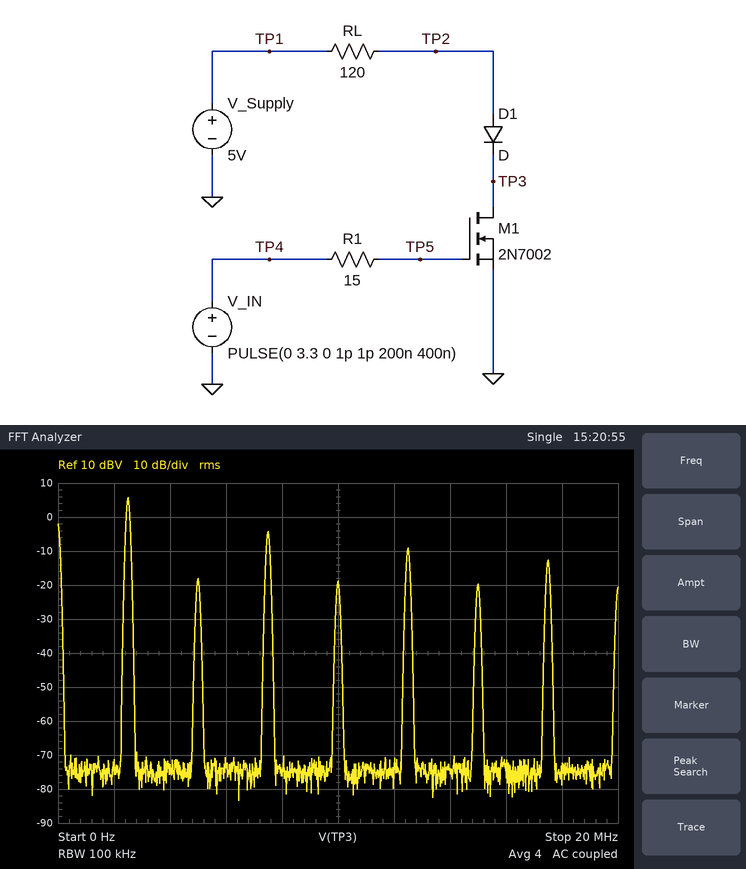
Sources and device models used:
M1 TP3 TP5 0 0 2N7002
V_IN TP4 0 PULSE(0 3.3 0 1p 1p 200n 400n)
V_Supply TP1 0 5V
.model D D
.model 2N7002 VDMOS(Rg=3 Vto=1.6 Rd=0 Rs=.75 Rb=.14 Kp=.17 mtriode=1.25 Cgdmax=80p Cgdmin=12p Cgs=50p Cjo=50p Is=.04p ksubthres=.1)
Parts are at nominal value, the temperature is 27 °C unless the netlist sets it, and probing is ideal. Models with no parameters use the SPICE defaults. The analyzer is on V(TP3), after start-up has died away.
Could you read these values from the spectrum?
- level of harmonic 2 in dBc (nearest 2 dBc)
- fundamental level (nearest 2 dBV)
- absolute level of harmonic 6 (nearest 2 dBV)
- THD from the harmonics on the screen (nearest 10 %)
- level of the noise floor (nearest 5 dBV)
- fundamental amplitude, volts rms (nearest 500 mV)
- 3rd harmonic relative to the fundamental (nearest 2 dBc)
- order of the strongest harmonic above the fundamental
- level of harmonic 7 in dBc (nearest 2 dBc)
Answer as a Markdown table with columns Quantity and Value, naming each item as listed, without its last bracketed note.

| Quantity | Value |
|---|---|
| level of harmonic 2 in dBc | -24 dBc |
| fundamental level | 6 dBV |
| absolute level of harmonic 6 | -20 dBV |
| THD from the harmonics on the screen | 40 % |
| level of the noise floor | -75 dBV |
| fundamental amplitude, volts rms | 2.0 V |
| 3rd harmonic relative to the fundamental | -10 dBc |
| order of the strongest harmonic above the fundamental | 3 |
| level of harmonic 7 in dBc | -18 dBc |
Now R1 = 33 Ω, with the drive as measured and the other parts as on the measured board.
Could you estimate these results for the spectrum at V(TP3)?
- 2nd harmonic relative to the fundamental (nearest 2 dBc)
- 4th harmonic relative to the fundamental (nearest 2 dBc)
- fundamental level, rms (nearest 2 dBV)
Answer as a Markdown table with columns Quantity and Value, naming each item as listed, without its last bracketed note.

| Quantity | Value |
|---|---|
| 2nd harmonic relative to the fundamental | -26 dBc |
| 4th harmonic relative to the fundamental | -28 dBc |
| fundamental level, rms | 6 dBV |
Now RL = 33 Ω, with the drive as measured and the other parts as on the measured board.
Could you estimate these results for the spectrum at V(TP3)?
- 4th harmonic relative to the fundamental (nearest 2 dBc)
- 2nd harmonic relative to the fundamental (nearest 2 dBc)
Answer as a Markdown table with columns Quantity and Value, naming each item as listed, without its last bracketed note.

| Quantity | Value |
|---|---|
| 4th harmonic relative to the fundamental | -40 dBc |
| 2nd harmonic relative to the fundamental | -40 dBc |
